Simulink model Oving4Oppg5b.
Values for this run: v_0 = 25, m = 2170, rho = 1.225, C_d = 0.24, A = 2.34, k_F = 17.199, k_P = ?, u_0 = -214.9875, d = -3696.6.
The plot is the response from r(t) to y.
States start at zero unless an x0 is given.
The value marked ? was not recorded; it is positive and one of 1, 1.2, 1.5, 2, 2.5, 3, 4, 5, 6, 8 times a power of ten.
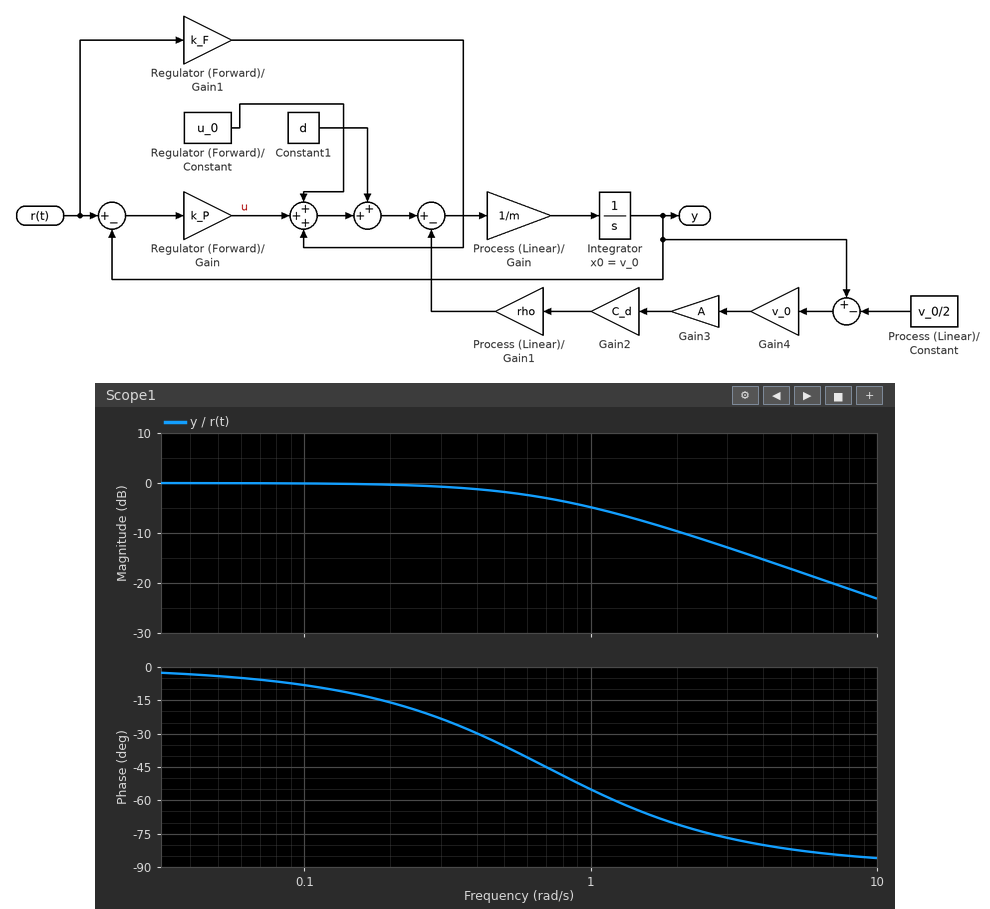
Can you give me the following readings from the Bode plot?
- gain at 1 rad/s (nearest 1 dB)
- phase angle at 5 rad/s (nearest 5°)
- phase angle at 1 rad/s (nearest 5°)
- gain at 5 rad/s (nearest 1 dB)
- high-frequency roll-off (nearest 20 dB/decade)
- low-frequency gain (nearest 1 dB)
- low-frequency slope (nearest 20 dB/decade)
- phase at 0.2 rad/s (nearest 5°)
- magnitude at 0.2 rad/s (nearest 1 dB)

-5 dB
-80°
-55°
-17 dB
-20 dB/decade
0 dB
0 dB/decade
-15°
0 dB
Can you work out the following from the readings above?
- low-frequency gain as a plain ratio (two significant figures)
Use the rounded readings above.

1.0
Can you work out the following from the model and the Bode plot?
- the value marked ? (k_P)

1500
